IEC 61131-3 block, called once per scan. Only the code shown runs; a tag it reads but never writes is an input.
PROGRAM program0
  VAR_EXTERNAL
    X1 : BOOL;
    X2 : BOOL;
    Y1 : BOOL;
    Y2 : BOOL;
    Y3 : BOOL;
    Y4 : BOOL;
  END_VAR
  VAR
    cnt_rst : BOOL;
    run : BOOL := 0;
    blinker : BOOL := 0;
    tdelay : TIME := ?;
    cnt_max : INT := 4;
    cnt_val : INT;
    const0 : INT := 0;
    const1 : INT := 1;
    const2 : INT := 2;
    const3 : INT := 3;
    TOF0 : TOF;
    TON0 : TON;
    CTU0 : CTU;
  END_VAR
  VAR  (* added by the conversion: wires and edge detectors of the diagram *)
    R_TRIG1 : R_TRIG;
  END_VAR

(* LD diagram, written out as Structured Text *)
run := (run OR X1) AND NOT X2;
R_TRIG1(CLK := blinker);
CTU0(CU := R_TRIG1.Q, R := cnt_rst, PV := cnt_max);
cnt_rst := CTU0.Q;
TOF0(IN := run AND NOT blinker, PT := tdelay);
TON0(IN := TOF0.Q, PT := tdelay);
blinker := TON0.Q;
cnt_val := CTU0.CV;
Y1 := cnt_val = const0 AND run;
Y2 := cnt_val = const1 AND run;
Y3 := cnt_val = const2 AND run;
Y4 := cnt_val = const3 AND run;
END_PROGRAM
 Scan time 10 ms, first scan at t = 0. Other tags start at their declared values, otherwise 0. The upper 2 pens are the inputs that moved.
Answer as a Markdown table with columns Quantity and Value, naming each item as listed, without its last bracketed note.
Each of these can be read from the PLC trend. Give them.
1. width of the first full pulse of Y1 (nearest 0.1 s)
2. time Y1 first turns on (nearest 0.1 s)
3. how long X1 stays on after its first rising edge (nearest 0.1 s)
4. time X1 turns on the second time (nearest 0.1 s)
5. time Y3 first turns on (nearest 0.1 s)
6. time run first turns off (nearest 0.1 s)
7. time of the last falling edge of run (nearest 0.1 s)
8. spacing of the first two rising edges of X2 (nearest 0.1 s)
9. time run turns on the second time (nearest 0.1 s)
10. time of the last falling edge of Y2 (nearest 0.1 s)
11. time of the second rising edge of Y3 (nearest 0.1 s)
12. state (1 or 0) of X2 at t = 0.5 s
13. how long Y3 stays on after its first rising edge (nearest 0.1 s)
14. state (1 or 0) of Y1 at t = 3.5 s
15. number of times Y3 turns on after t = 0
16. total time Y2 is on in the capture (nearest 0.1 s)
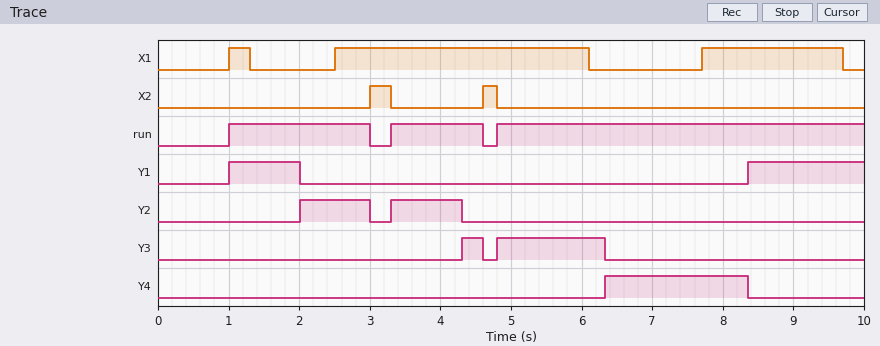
| Quantity | Value |
|---|---|
| width of the first full pulse of Y1 | 1.0 s |
| time Y1 first turns on | 1.0 s |
| how long X1 stays on after its first rising edge | 0.3 s |
| time X1 turns on the second time | 2.5 s |
| time Y3 first turns on | 4.3 s |
| time run first turns off | 3.0 s |
| time of the last falling edge of run | 4.6 s |
| spacing of the first two rising edges of X2 | 1.6 s |
| time run turns on the second time | 3.3 s |
| time of the last falling edge of Y2 | 4.3 s |
| time of the second rising edge of Y3 | 4.8 s |
| state (1 or 0) of X2 at t = 0.5 s | 0 |
| how long Y3 stays on after its first rising edge | 0.3 s |
| state (1 or 0) of Y1 at t = 3.5 s | 0 |
| number of times Y3 turns on after t = 0 | 2 |
| total time Y2 is on in the capture | 2.0 s |
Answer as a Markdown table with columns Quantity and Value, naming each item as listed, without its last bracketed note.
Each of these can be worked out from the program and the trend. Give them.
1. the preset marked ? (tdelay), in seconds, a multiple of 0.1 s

| Quantity | Value |
|---|---|
| the preset marked ? (tdelay), in seconds, a multiple of 0.1 s | 1.0 s |
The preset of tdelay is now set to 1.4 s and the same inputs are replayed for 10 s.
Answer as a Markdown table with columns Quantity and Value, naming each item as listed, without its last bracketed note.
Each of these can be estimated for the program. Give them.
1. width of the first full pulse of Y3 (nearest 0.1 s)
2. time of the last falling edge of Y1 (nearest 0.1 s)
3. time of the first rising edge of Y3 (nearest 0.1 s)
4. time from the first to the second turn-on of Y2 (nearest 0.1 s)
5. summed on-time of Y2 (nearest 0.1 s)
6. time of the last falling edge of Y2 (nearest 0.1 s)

| Quantity | Value |
|---|---|
| width of the first full pulse of Y3 | 2.8 s |
| time of the last falling edge of Y1 | 2.4 s |
| time of the first rising edge of Y3 | 5.2 s |
| time from the first to the second turn-on of Y2 | 0.9 s |
| summed on-time of Y2 | 2.3 s |
| time of the last falling edge of Y2 | 5.2 s |
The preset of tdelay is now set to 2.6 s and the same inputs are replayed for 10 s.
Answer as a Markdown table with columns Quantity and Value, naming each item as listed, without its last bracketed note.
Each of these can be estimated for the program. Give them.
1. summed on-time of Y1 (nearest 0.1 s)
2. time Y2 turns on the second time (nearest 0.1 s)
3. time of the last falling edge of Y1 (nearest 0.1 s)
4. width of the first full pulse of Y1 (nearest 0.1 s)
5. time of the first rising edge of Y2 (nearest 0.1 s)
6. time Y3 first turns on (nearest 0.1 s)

| Quantity | Value |
|---|---|
| summed on-time of Y1 | 2.3 s |
| time Y2 turns on the second time | 4.8 s |
| time of the last falling edge of Y1 | 3.6 s |
| width of the first full pulse of Y1 | 2.0 s |
| time of the first rising edge of Y2 | 3.6 s |
| time Y3 first turns on | 8.8 s |
